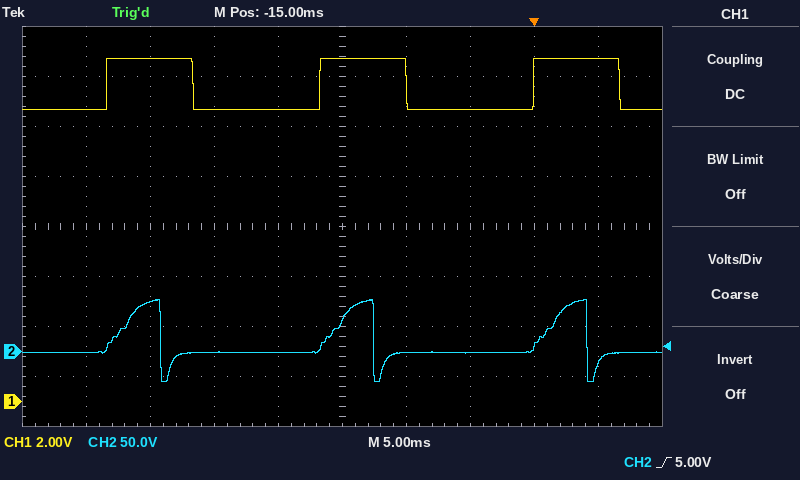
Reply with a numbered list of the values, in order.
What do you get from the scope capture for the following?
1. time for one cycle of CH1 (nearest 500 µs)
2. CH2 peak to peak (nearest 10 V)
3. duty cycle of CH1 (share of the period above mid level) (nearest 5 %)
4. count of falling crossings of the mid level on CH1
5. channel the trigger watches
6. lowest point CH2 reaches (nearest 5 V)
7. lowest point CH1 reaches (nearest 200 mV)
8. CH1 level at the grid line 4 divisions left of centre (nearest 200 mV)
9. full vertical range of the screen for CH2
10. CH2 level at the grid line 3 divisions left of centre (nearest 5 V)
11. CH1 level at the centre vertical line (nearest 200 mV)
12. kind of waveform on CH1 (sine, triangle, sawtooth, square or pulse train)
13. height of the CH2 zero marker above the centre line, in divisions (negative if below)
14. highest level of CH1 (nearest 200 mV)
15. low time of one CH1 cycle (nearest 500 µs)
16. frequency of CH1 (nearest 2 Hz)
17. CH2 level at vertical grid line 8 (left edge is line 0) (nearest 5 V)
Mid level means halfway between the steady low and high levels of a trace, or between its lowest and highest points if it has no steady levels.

1. 16.5 ms
2. 80 V
3. 40 %
4. 3
5. CH2
6. -30 V
7. 11.6 V
8. 11.6 V
9. 400 V
10. 50 V
11. 13.8 V
12. pulse train
13. -2.5 div
14. 13.8 V
15. 10.0 ms
16. 60 Hz
17. 5 V
